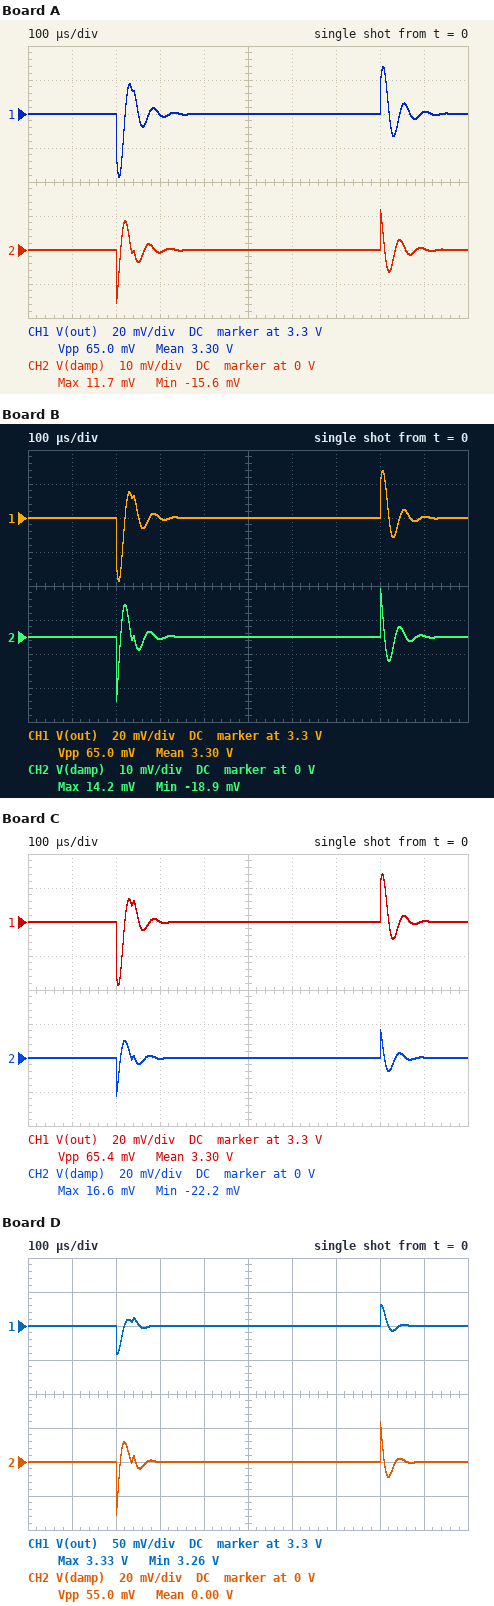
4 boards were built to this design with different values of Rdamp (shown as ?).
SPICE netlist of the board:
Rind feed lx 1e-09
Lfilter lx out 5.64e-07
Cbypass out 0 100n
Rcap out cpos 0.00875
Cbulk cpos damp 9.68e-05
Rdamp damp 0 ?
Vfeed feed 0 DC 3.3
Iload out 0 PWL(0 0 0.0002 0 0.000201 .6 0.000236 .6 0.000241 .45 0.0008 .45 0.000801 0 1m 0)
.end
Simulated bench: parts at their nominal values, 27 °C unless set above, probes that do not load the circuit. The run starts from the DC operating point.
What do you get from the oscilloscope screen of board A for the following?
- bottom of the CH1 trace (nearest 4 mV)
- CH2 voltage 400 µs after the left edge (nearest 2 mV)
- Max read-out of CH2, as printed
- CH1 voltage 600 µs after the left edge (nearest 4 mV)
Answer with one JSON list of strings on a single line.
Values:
["3.264 V", "0 V", "11.7 mV", "3.300 V"]
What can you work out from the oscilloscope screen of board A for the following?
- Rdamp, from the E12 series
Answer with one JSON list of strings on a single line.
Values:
["0.027 Ω"]
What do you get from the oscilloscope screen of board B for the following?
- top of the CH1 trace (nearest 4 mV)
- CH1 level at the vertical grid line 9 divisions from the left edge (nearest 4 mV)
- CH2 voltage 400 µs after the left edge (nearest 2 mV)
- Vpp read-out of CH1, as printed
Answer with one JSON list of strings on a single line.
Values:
["3.328 V", "3.300 V", "0 V", "65.0 mV"]
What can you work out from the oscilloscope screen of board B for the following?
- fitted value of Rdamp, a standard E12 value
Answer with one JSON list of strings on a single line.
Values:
["0.033 Ω"]
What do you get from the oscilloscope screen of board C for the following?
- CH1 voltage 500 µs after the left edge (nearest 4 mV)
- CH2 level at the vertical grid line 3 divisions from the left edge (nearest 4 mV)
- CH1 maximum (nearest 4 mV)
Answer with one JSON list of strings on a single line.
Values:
["3.300 V", "0 V", "3.328 V"]
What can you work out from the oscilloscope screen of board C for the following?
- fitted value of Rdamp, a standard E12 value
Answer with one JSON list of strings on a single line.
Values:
["0.039 Ω"]
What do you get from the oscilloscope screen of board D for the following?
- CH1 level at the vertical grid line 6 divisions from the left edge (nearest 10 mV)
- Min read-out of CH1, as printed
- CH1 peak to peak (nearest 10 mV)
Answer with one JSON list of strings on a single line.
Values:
["3.30 V", "3.26 V", "70 mV"]
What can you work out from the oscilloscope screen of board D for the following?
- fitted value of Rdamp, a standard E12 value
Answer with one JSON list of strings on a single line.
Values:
["0.056 Ω"]
